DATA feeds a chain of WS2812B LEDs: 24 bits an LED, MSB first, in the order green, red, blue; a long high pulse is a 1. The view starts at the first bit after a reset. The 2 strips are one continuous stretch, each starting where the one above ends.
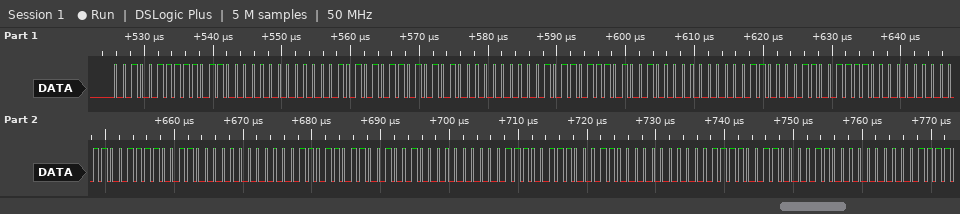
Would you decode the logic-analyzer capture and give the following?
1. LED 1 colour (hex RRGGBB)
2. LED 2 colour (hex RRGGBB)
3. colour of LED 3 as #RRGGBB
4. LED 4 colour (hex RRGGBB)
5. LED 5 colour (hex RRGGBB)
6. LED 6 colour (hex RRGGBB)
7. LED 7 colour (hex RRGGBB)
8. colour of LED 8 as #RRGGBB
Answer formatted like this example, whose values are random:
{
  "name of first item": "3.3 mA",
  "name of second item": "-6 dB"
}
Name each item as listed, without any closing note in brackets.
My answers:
{
  "LED 1 colour": "#D82700",
  "LED 2 colour": "#D52A00",
  "colour of LED 3 as #RRGGBB": "#D22D00",
  "LED 4 colour": "#CF3000",
  "LED 5 colour": "#CC3300",
  "LED 6 colour": "#C93600",
  "LED 7 colour": "#C63900",
  "colour of LED 8 as #RRGGBB": "#C33C00"
}
